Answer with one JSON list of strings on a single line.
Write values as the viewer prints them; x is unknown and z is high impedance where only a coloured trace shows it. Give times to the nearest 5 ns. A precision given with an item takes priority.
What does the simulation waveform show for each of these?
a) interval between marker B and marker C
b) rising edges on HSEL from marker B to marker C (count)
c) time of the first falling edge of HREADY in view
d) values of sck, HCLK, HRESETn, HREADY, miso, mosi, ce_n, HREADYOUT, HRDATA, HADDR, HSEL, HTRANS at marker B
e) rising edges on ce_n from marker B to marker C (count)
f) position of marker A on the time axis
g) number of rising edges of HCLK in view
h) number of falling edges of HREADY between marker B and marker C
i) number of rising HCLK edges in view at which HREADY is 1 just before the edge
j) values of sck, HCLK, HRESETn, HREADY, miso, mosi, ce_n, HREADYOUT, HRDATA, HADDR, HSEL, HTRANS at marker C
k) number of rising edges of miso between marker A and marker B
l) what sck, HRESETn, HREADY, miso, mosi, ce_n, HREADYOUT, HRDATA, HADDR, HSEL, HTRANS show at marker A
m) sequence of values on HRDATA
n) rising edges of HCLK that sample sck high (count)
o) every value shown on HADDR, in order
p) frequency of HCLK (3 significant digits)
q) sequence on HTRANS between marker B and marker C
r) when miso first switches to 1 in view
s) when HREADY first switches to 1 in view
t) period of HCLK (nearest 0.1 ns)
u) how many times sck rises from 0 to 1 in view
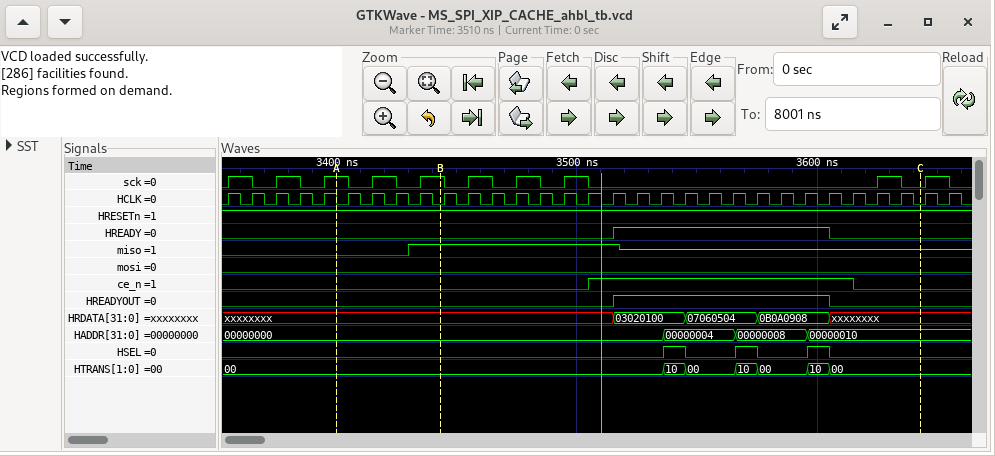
["200 ns", "3", "3605 ns", "sck=1, HCLK=0, HRESETn=1, HREADY=0, miso=1, mosi=0, ce_n=0, HREADYOUT=0, HRDATA=xxxxxxxx, HADDR=00000000, HSEL=0, HTRANS=00", "1", "3400 ns", "31", "1", "9", "sck=0, HCLK=0, HRESETn=1, HREADY=0, miso=z, mosi=0, ce_n=0, HREADYOUT=0, HRDATA=xxxxxxxx, HADDR=00000010, HSEL=0, HTRANS=00", "1", "sck=1, HRESETn=1, HREADY=0, miso=0, mosi=0, ce_n=0, HREADYOUT=0, HRDATA=xxxxxxxx, HADDR=00000000, HSEL=0, HTRANS=00", "xxxxxxxx, 03020100, 07060504, 0B0A0908, xxxxxxxx", "10", "00000000, 00000004, 00000008, 00000010", "100 MHz", "00, 10, 00, 10, 00, 10, 00", "3430 ns", "3515 ns", "10 ns", "10"]
